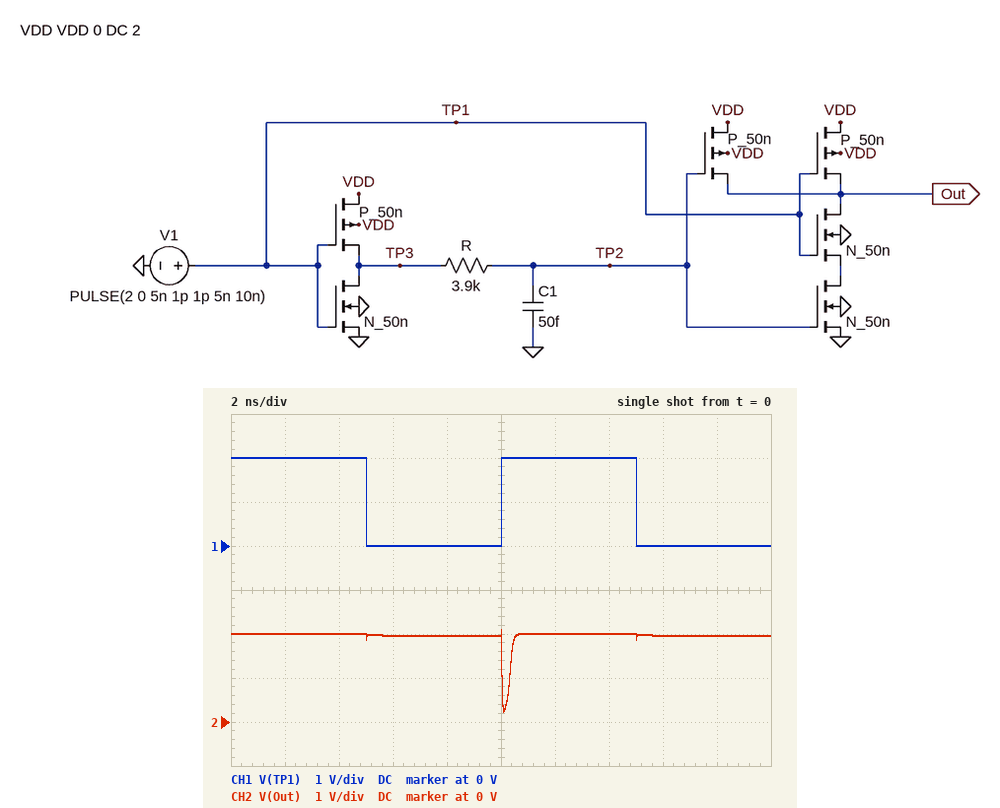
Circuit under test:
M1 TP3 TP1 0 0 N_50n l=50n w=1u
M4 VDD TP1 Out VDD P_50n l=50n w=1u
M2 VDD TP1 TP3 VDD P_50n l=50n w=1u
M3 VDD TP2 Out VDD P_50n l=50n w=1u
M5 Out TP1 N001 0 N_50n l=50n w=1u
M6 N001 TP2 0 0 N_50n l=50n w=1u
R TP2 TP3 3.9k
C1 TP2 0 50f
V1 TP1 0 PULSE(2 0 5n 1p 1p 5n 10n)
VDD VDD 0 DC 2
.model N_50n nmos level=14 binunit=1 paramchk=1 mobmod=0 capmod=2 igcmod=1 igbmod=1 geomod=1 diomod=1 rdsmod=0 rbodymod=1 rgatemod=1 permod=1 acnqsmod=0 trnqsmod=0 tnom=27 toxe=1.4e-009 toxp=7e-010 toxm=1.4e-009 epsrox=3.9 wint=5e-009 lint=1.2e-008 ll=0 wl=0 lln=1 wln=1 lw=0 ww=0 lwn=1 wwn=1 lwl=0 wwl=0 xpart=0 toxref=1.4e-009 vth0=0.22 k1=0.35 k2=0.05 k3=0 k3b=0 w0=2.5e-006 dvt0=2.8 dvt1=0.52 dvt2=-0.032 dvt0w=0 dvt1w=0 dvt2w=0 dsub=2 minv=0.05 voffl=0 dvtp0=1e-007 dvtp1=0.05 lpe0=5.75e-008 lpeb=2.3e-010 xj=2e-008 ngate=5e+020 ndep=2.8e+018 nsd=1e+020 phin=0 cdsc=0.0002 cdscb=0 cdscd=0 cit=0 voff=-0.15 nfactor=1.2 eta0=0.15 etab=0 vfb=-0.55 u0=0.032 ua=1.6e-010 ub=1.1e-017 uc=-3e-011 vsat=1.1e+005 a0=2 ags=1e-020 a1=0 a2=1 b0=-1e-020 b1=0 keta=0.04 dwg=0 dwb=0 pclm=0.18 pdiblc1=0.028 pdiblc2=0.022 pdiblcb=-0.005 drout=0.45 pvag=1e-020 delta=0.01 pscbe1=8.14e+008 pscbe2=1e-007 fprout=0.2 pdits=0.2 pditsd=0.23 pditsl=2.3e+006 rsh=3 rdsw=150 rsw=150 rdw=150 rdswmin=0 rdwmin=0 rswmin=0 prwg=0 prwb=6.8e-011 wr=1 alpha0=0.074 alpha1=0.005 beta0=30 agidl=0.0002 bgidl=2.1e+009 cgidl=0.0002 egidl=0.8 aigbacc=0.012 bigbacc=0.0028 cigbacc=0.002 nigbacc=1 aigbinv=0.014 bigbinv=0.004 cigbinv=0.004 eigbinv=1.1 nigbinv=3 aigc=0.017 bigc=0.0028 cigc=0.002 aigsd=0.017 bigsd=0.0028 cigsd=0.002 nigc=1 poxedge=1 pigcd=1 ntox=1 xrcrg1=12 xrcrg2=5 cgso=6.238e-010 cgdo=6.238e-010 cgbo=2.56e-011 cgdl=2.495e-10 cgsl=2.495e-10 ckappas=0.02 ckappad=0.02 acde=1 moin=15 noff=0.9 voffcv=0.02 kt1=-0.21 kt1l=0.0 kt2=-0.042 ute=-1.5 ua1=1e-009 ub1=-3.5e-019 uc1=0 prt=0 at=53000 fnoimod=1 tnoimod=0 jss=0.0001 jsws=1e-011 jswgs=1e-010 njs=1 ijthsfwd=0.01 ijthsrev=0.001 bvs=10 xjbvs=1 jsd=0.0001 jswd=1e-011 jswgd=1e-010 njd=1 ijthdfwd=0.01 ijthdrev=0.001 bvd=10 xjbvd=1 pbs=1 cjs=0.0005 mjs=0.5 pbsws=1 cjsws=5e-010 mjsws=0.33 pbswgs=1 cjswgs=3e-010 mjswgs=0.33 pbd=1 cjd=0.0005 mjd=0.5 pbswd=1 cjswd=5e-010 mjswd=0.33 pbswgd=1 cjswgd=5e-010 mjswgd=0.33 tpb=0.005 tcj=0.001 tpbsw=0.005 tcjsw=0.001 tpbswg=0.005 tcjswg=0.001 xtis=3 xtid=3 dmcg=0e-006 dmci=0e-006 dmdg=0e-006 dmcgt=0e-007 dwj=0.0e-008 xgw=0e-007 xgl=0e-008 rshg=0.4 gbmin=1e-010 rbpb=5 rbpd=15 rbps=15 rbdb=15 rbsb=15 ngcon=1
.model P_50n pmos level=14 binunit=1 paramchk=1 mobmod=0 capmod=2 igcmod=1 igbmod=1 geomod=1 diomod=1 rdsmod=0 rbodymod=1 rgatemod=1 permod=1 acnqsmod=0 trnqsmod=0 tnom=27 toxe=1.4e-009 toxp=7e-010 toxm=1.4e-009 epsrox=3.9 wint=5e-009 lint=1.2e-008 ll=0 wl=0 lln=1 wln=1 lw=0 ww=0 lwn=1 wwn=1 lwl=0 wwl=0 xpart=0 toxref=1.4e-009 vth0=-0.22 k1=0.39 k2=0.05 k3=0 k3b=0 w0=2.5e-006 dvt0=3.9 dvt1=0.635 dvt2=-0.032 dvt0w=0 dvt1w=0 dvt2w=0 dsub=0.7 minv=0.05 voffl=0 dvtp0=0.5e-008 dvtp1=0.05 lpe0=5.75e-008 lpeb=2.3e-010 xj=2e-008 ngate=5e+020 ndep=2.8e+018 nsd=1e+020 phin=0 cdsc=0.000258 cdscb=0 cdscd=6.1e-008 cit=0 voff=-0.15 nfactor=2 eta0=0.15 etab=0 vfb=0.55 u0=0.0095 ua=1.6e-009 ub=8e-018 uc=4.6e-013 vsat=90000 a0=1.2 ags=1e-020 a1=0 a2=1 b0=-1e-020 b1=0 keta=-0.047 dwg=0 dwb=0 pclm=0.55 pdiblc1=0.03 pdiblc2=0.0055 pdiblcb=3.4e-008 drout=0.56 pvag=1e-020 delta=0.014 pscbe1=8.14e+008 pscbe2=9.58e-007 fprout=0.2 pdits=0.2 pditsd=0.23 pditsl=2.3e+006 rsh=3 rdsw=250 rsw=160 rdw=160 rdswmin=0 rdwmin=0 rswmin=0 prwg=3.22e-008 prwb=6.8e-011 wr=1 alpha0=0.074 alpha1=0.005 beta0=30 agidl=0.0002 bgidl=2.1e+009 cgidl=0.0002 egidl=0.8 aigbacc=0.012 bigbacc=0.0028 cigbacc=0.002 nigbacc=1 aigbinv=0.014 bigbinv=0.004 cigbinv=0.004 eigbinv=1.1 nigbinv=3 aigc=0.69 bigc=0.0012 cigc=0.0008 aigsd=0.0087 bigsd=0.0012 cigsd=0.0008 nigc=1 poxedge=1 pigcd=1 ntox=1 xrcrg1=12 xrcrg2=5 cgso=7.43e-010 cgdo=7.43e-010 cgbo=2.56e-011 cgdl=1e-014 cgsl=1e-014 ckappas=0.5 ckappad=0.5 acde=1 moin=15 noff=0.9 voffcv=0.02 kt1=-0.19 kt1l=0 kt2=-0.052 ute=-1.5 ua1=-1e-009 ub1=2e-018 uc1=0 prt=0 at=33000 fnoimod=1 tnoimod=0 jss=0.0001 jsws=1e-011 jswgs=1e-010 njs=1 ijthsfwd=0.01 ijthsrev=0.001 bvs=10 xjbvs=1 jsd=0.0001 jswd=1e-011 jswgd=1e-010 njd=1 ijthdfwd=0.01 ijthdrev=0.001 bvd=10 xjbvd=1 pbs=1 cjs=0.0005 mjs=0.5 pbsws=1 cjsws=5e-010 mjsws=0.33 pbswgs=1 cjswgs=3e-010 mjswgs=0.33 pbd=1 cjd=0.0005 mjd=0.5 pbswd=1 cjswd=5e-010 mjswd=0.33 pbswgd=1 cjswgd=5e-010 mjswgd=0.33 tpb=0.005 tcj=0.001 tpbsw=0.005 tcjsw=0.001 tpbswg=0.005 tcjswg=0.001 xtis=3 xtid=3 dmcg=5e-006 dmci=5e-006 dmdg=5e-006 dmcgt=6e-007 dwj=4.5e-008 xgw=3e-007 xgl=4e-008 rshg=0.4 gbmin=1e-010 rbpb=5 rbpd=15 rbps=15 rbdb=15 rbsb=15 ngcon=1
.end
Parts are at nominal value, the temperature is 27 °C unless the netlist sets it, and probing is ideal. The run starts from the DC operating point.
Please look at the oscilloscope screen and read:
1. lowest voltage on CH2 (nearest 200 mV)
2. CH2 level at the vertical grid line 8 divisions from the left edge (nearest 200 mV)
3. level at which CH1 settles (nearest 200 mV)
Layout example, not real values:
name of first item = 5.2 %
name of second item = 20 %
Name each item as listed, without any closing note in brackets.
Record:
lowest voltage on CH2 = 200 mV
CH2 level at the vertical grid line 8 divisions from the left edge = 2.0 V
level at which CH1 settles = 0 V
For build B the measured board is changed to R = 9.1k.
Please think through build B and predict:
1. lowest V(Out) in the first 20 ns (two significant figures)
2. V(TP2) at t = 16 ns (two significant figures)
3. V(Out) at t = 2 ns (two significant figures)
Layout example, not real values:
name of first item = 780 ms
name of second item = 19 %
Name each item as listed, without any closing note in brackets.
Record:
lowest V(Out) in the first 20 ns = 120 mV
V(TP2) at t = 16 ns = 1.6 V
V(Out) at t = 2 ns = 2.0 V
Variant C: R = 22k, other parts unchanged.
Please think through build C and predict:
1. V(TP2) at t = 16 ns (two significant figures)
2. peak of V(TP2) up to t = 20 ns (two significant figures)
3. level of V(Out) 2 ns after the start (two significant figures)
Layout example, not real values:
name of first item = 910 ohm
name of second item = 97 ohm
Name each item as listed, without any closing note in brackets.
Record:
V(TP2) at t = 16 ns = 1.1 V
peak of V(TP2) up to t = 20 ns = 1.9 V
level of V(Out) 2 ns after the start = 2.0 V
